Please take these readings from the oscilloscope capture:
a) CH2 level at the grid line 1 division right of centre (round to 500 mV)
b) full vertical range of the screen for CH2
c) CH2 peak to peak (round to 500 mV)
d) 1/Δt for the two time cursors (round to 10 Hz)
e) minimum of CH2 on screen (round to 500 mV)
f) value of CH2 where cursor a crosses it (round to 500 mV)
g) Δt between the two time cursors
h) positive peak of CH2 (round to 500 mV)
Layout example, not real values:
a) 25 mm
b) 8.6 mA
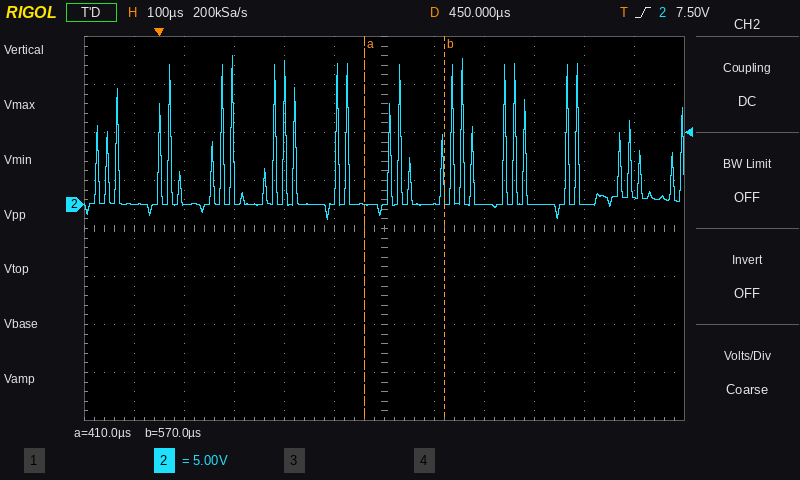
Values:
a) 0.0 V
b) 40 V
c) 17.0 V
d) 6.25 kHz
e) -1.5 V
f) 0.0 V
g) 160 µs
h) 15.5 V
